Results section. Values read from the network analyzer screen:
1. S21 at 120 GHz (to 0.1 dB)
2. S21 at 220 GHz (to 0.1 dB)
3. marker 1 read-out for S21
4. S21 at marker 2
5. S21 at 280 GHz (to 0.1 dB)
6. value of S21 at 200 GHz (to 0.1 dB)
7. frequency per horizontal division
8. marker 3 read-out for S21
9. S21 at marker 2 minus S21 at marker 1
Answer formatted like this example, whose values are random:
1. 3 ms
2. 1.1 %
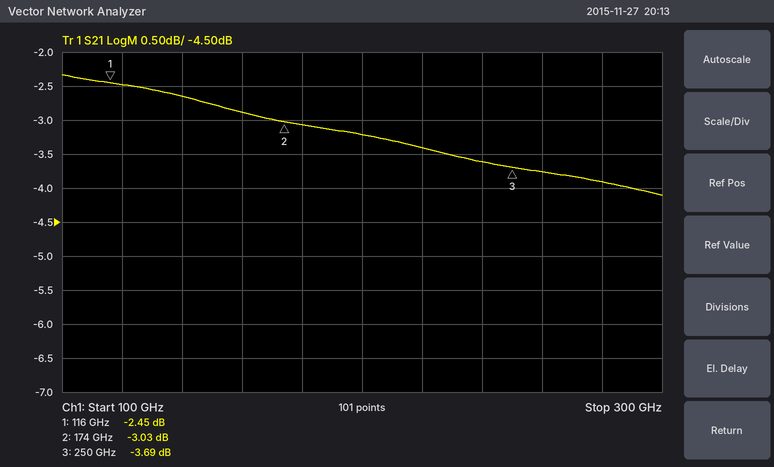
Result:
1. -2.5 dB
2. -3.4 dB
3. -2.45 dB
4. -3.03 dB
5. -3.9 dB
6. -3.2 dB
7. 20 GHz
8. -3.69 dB
9. -0.58 dB
